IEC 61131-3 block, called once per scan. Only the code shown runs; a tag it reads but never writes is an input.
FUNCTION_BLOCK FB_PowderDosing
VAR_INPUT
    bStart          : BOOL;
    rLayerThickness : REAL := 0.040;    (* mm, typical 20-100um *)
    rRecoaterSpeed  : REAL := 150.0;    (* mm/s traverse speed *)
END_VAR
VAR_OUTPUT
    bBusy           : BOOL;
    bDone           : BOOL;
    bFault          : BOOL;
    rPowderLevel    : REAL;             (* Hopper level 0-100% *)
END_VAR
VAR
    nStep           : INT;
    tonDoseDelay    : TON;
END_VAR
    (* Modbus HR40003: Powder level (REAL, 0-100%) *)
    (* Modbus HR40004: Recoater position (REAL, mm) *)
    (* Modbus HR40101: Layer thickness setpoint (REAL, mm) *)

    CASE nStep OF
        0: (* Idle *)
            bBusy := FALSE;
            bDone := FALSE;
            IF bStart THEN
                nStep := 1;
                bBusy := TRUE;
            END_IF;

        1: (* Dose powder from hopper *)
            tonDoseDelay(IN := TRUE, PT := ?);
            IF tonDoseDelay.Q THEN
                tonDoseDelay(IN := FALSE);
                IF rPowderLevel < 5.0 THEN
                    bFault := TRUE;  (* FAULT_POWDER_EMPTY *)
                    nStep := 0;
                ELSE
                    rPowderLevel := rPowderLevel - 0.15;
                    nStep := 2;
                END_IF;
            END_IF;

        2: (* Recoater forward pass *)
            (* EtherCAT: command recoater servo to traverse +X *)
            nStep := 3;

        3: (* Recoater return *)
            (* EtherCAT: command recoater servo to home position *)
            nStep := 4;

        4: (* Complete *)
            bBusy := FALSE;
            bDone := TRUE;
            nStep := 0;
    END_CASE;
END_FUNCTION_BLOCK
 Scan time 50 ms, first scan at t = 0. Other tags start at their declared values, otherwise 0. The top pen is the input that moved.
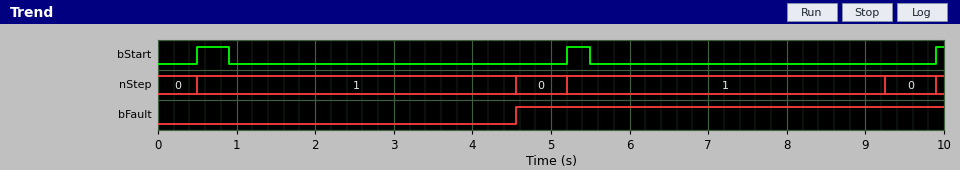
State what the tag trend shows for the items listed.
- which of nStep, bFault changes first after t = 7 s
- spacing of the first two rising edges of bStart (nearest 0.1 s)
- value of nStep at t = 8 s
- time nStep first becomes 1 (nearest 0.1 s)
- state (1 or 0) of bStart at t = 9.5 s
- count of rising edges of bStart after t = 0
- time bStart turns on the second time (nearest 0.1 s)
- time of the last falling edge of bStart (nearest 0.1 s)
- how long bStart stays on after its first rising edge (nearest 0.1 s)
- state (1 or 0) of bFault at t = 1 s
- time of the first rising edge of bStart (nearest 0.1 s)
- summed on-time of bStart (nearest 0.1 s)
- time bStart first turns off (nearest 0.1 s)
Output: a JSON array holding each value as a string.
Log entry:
["nStep", "4.7 s", "1", "0.5 s", "0", "3", "5.2 s", "5.5 s", "0.4 s", "0", "0.5 s", "0.8 s", "0.9 s"]
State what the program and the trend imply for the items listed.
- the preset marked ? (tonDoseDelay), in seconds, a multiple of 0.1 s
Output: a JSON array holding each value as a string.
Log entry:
["4.0 s"]
